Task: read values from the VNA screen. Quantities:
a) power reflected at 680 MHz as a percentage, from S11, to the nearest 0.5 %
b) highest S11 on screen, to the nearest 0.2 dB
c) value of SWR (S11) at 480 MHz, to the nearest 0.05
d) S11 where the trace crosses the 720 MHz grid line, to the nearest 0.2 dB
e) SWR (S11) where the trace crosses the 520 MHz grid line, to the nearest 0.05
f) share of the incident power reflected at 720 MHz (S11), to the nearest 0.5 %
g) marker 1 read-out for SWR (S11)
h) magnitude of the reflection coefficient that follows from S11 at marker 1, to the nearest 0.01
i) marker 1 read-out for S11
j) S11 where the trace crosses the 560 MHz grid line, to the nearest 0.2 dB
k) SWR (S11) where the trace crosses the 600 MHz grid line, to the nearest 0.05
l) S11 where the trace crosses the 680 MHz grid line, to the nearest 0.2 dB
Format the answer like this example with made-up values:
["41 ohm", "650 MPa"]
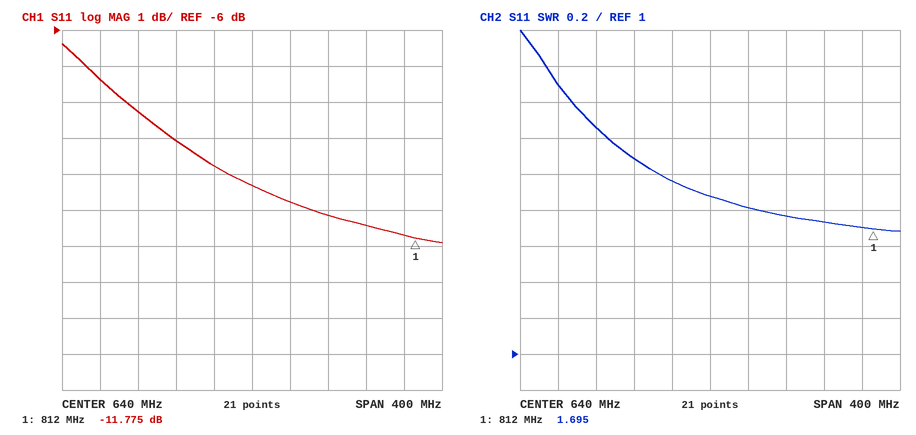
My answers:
["8.5 %", "-6.4 dB", "2.50", "-11.2 dB", "2.25", "7.5 %", "1.695", "0.26", "-11.775 dB", "-9.0 dB", "1.95", "-10.8 dB"]
